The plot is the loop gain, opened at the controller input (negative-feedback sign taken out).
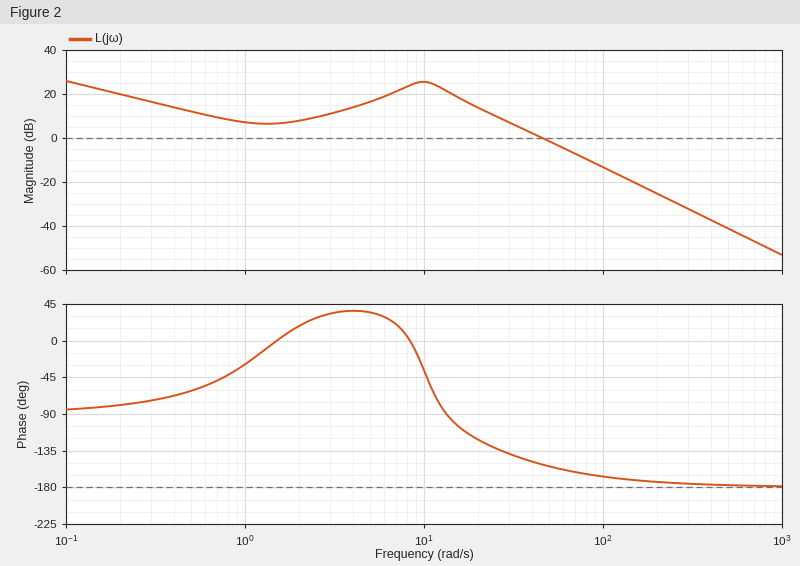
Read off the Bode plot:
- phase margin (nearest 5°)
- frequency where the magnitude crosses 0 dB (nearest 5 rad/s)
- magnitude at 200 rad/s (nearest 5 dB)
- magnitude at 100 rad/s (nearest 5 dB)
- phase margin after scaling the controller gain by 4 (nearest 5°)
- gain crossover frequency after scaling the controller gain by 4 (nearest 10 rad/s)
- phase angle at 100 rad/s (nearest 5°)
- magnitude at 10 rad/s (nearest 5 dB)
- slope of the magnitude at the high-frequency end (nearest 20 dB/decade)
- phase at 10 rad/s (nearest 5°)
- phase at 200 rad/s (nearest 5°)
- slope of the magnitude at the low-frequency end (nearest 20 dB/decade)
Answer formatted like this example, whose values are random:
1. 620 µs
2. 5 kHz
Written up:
1. 30°
2. 45 rad/s
3. -25 dB
4. -15 dB
5. 15°
6. 90 rad/s
7. -165°
8. 25 dB
9. -40 dB/decade
10. -35°
11. -175°
12. -20 dB/decade
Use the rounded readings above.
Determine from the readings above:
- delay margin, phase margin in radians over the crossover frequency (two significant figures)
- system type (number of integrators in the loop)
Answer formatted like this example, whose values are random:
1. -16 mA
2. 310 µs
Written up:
1. 0.012 s
2. 1
